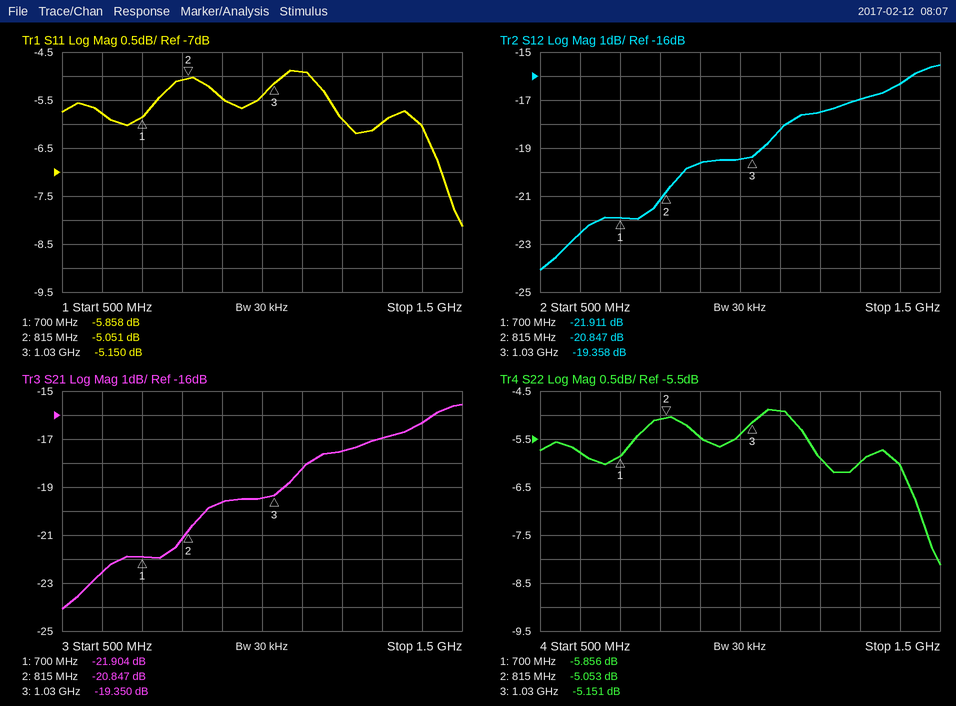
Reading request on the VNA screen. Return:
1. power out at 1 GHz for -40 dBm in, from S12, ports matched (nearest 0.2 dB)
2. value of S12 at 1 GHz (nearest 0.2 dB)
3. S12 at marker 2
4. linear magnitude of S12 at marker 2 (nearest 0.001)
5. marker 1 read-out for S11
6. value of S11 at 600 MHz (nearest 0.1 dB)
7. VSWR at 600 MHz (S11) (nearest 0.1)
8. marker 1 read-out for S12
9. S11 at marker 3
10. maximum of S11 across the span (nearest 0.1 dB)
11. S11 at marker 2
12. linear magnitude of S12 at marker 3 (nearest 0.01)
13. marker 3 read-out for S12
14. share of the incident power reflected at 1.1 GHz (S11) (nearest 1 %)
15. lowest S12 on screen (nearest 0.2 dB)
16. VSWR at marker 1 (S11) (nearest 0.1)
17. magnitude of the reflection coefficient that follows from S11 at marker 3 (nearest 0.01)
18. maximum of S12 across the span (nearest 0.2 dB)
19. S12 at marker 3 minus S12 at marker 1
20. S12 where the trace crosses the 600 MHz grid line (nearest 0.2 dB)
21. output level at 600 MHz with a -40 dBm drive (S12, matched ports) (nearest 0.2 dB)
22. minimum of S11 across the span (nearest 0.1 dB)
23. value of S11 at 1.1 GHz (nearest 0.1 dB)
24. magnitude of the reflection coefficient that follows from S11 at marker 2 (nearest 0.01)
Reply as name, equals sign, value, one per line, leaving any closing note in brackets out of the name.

power out at 1 GHz for -40 dBm in, from S12, ports matched = -59.4 dBm
value of S12 at 1 GHz = -19.4 dB
S12 at marker 2 = -20.847 dB
linear magnitude of S12 at marker 2 = 0.091
marker 1 read-out for S11 = -5.858 dB
value of S11 at 600 MHz = -5.8 dB
VSWR at 600 MHz (S11) = 3.1
marker 1 read-out for S12 = -21.911 dB
S11 at marker 3 = -5.150 dB
maximum of S11 across the span = -4.9 dB
S11 at marker 2 = -5.051 dB
linear magnitude of S12 at marker 3 = 0.11
marker 3 read-out for S12 = -19.358 dB
share of the incident power reflected at 1.1 GHz (S11) = 32 %
lowest S12 on screen = -24.0 dB
VSWR at marker 1 (S11) = 3.1
magnitude of the reflection coefficient that follows from S11 at marker 3 = 0.55
maximum of S12 across the span = -15.6 dB
S12 at marker 3 minus S12 at marker 1 = 2.553 dB
S12 where the trace crosses the 600 MHz grid line = -22.6 dB
output level at 600 MHz with a -40 dBm drive (S12, matched ports) = -62.6 dBm
minimum of S11 across the span = -8.1 dB
value of S11 at 1.1 GHz = -4.9 dB
magnitude of the reflection coefficient that follows from S11 at marker 2 = 0.56
